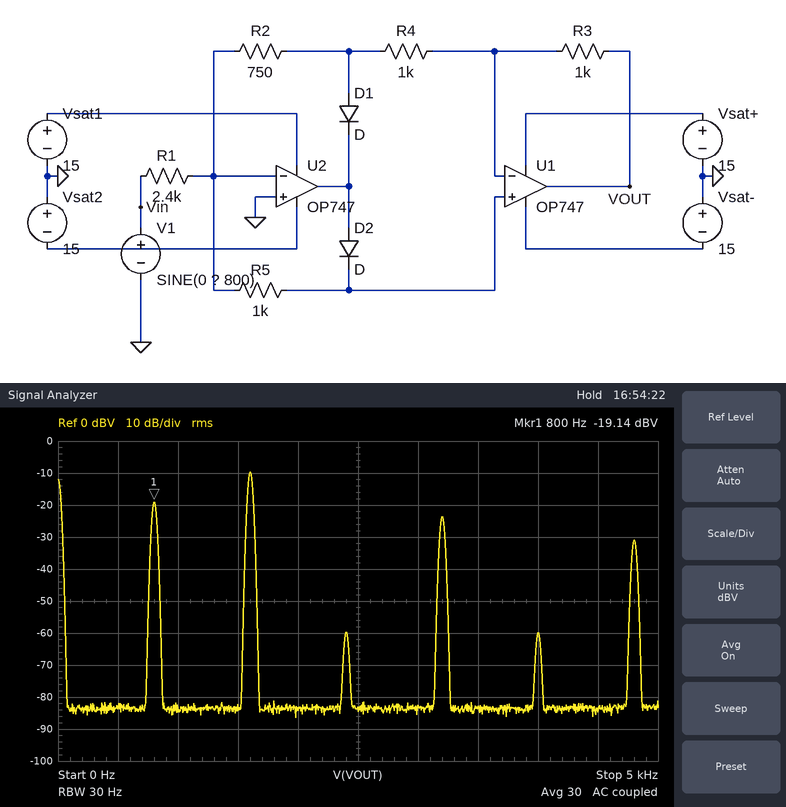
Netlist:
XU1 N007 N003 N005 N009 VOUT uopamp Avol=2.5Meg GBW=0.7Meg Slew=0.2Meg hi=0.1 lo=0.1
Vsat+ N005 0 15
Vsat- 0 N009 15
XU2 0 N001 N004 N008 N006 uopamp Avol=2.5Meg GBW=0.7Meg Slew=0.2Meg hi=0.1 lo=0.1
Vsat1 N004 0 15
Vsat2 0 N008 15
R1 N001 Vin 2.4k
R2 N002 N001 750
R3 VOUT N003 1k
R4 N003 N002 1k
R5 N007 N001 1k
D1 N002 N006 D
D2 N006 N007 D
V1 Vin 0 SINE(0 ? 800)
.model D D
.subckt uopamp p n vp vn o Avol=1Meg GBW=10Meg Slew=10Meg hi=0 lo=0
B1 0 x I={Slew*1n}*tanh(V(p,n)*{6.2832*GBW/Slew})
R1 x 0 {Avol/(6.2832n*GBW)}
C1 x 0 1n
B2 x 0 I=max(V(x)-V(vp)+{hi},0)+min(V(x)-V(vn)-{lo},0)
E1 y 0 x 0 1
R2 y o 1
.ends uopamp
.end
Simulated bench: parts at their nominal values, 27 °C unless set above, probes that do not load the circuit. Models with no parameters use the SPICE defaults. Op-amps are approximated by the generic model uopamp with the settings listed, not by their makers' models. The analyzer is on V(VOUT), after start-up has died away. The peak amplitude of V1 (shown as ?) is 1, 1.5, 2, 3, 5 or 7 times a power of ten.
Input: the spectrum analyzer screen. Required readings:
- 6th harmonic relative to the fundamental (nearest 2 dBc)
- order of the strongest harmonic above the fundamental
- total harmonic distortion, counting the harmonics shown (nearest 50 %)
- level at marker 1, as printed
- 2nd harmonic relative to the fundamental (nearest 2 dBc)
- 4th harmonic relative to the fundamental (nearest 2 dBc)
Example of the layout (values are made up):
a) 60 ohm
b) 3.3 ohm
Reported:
a) -12 dBc
b) 2
c) 300 %
d) -19.14 dBV
e) 10 dBc
f) -4 dBc
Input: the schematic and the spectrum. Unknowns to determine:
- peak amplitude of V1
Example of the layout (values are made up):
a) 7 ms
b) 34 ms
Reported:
a) 3 V
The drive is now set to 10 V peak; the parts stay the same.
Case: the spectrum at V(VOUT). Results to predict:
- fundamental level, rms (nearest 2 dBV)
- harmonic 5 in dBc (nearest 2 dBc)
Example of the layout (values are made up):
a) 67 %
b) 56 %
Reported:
a) -8 dBV
b) -46 dBc
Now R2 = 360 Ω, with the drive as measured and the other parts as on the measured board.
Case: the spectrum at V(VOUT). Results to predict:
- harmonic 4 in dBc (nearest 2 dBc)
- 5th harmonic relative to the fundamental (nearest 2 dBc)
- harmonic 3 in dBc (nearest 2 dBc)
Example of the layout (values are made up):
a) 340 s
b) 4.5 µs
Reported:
a) -14 dBc
b) -48 dBc
c) -48 dBc
